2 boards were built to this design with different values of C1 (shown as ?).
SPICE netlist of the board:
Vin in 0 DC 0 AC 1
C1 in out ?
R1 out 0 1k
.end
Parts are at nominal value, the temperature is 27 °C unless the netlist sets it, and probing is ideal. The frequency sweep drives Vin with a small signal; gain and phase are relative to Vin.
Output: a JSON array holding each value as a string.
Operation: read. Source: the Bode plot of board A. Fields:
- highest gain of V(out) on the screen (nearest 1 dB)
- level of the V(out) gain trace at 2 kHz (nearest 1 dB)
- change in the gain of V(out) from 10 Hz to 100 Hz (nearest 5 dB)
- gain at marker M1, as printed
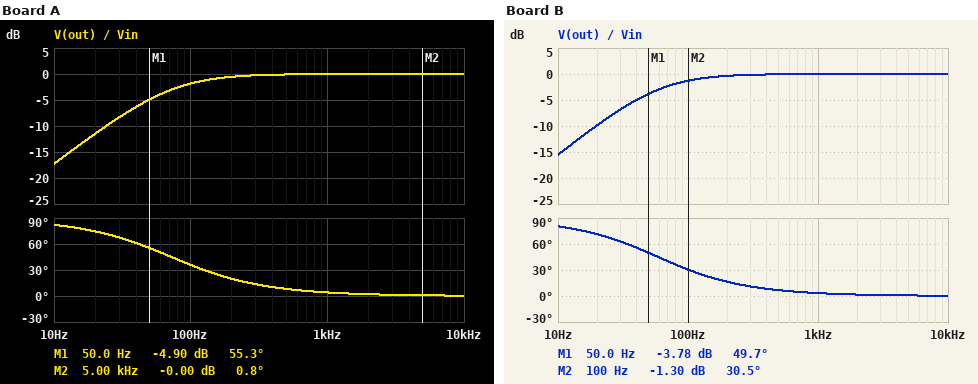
["0 dB", "0 dB", "15 dB", "-4.90 dB"]
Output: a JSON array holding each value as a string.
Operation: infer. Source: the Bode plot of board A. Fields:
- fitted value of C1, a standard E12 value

["2.2 µF"]
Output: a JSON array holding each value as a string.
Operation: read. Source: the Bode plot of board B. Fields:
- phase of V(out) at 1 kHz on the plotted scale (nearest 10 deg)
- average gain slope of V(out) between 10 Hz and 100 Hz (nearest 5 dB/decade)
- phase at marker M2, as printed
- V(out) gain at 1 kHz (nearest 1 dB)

["0 deg", "15 dB/decade", "30.5 deg", "0 dB"]
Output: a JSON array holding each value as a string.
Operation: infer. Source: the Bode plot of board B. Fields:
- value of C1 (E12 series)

["2.7 µF"]
